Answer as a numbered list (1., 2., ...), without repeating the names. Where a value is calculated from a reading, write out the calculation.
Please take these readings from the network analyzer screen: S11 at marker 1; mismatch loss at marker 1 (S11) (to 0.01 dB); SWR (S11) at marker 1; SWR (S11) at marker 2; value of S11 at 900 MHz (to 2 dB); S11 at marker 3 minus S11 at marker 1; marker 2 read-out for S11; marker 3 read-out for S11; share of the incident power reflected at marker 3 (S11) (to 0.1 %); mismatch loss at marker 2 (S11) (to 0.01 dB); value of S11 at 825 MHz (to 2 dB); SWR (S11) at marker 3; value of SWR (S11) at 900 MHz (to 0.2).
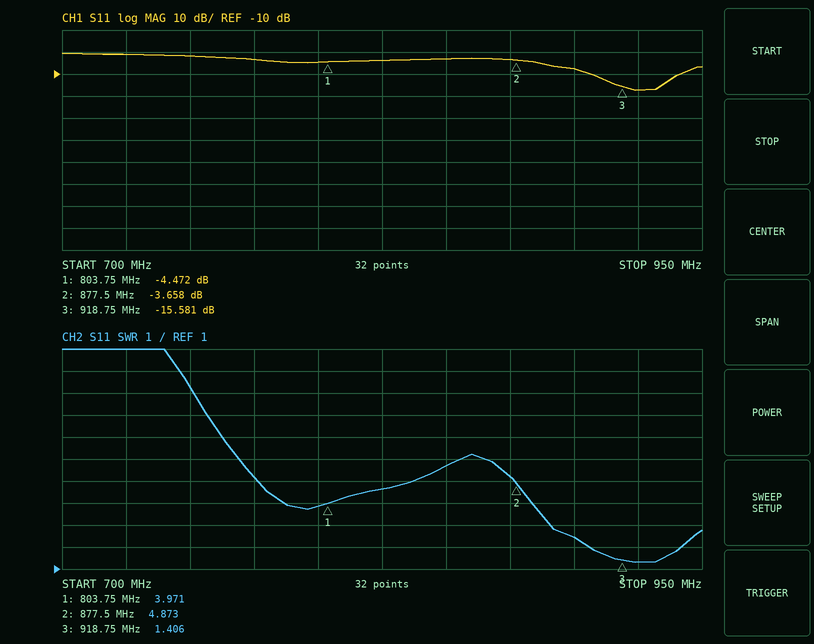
1. -4.472 dB
2. −10 log10(1 − 10^(-4.472/10)) ≈ 1.92 dB
3. 3.971
4. 4.873
5. -8 dB
6. -15.581 − (-4.472) = -11.109 dB
7. -3.658 dB
8. -15.581 dB
9. 10^(-15.581/10) ≈ 2.8 %
10. −10 log10(1 − 10^(-3.658/10)) ≈ 2.45 dB
11. -4 dB
12. 1.406
13. 2.4
